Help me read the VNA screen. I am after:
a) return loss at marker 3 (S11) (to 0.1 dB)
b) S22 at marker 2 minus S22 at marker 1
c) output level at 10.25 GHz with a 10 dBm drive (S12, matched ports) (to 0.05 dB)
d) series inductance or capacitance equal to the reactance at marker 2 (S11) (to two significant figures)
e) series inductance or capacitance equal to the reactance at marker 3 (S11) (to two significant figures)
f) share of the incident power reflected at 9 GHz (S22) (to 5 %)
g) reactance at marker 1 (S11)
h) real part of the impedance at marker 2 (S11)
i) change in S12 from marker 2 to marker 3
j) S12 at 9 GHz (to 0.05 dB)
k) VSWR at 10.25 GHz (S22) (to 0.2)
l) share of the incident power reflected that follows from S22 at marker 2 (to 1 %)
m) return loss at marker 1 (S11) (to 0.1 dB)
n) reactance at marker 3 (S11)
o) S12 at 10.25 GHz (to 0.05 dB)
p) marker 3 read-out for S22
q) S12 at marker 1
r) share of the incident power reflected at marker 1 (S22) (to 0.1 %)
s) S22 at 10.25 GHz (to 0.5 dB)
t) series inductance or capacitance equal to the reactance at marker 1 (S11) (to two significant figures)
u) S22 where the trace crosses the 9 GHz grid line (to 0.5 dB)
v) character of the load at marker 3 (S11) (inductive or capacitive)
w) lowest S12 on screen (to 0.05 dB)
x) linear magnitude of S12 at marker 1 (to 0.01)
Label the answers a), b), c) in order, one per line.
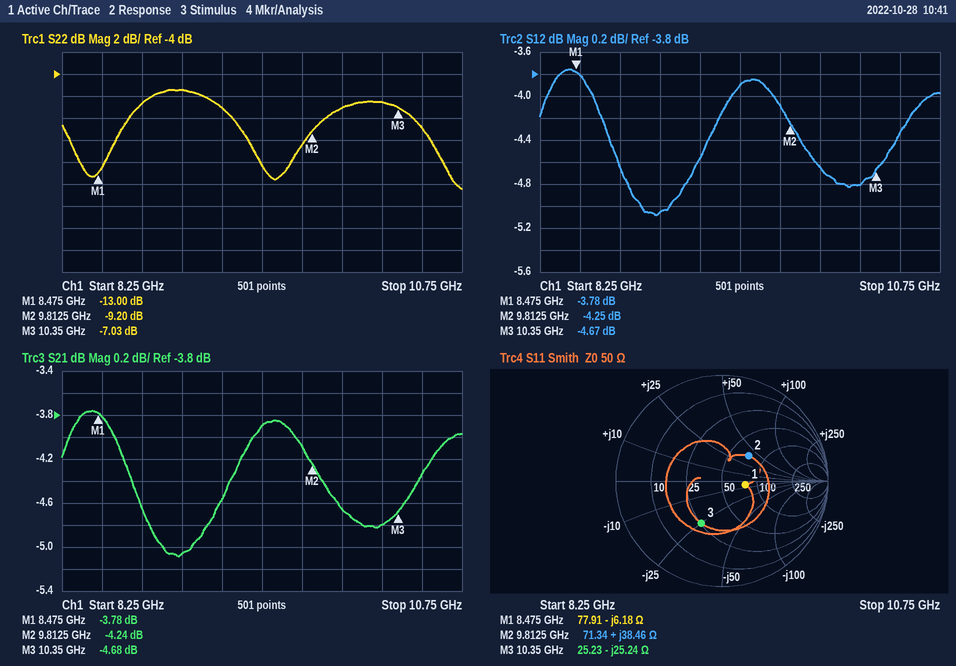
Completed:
a) 7.0 dB
b) 3.80 dB
c) 5.20 dBm
d) 620 pH
e) 610 fF
f) 30 %
g) -6.18 Ω
h) 71.34 Ω
i) -0.42 dB
j) -5.05 dB
k) 2.8
l) 12 %
m) 13.0 dB
n) -25.24 Ω
o) -4.80 dB
p) -7.03 dB
q) -3.78 dB
r) 5.0 %
s) -6.5 dB
t) 3.0 pF
u) -5.5 dB
v) capacitive
w) -5.10 dB
x) 0.65
